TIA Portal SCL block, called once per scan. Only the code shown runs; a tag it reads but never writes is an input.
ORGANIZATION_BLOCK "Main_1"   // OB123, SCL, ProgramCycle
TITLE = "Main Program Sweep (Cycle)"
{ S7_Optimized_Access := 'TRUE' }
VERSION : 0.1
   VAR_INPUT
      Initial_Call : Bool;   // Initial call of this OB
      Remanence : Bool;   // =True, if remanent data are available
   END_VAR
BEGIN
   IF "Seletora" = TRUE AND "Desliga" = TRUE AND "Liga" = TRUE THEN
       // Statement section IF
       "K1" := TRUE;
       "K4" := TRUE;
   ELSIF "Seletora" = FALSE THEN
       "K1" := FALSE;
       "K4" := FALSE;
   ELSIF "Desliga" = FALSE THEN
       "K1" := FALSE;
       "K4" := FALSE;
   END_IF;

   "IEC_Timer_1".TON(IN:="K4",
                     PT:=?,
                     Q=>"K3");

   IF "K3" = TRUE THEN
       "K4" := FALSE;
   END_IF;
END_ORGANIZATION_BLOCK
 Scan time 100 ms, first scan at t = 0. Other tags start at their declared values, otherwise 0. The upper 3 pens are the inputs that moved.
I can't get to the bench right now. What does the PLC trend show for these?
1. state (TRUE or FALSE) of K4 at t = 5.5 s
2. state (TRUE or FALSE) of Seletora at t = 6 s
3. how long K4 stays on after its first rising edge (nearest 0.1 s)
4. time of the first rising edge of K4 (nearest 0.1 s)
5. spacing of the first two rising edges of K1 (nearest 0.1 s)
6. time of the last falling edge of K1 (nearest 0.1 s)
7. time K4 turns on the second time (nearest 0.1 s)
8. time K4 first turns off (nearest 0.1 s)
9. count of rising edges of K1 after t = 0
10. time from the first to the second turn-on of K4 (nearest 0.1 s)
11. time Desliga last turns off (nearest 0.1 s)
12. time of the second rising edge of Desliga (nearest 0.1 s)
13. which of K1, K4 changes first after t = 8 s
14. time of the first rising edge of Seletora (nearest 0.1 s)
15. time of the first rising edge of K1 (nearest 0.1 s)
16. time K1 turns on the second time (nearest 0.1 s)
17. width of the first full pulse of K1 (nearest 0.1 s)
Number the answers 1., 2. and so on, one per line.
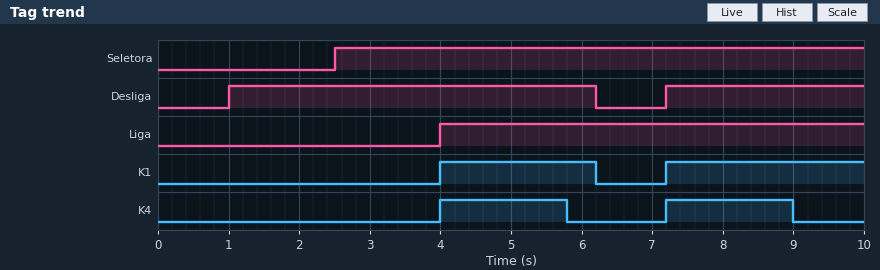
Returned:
1. TRUE
2. TRUE
3. 1.8 s
4. 4.0 s
5. 3.2 s
6. 6.2 s
7. 7.2 s
8. 5.8 s
9. 2
10. 3.2 s
11. 6.2 s
12. 7.2 s
13. K4
14. 2.5 s
15. 4.0 s
16. 7.2 s
17. 2.2 s
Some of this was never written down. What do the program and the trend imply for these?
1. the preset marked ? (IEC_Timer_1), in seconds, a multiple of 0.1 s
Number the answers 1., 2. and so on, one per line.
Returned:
1. 1.8 s
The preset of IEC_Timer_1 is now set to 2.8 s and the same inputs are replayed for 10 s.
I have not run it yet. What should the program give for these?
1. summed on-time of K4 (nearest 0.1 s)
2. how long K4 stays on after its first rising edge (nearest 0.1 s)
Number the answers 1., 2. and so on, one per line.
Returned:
1. 5.0 s
2. 2.2 s
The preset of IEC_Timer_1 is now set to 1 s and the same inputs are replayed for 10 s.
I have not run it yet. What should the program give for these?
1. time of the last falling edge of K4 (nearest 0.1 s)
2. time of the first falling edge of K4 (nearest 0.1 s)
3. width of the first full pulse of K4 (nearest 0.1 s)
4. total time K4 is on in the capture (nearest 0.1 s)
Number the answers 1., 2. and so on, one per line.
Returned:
1. 8.2 s
2. 5.0 s
3. 1.0 s
4. 2.0 s
